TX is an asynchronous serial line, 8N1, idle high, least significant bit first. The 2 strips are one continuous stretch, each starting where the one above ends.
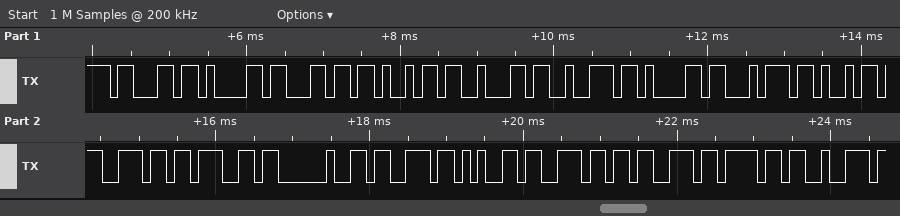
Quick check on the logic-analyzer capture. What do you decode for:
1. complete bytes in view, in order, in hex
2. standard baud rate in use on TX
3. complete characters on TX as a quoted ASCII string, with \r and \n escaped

0x63 0x61 0x6C 0x69 0x62 0x72 0x61 0x74 0x69 0x6E 0x67 0x20 0x73 0x65 0x6E 0x73 0x6F 0x72
9600 baud
"calibrating sensor"
